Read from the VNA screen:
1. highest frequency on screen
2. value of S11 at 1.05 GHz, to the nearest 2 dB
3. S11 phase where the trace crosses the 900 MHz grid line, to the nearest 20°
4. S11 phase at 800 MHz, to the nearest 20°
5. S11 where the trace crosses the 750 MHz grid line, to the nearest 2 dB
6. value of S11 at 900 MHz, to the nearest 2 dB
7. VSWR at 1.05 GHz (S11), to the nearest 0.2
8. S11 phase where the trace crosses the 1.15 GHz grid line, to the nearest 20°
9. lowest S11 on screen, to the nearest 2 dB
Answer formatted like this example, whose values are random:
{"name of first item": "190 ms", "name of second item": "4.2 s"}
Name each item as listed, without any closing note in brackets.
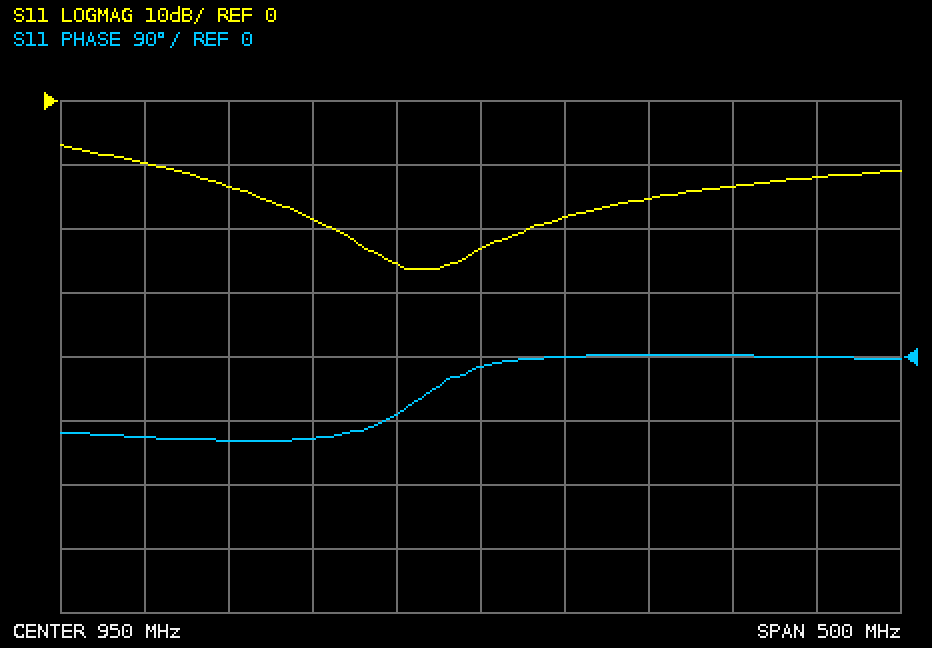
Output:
{"highest frequency on screen": "1.2 GHz", "value of S11 at 1.05 GHz, to the nearest 2 dB": "-16 dB", "S11 phase where the trace crosses the 900 MHz grid line, to the nearest 20°": "-80°", "S11 phase at 800 MHz, to the nearest 20°": "-120°", "S11 where the trace crosses the 750 MHz grid line, to the nearest 2 dB": "-10 dB", "value of S11 at 900 MHz, to the nearest 2 dB": "-26 dB", "VSWR at 1.05 GHz (S11), to the nearest 0.2": "1.4", "S11 phase where the trace crosses the 1.15 GHz grid line, to the nearest 20°": "0°", "lowest S11 on screen, to the nearest 2 dB": "-26 dB"}
